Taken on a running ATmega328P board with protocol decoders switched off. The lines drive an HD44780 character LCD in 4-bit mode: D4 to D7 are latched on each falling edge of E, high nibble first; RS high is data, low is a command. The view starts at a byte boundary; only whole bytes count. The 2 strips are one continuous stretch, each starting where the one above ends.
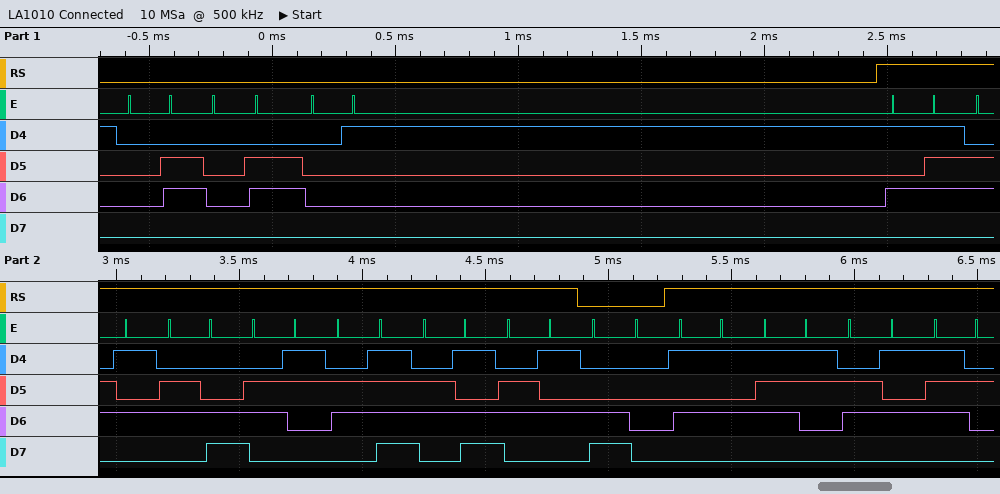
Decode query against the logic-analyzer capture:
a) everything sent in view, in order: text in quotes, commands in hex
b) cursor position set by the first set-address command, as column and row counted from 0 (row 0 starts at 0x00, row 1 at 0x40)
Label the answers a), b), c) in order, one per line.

a) 0x06 0x06 0x01 "Welcome" 0xC0 "User"
b) column 0, row 1
